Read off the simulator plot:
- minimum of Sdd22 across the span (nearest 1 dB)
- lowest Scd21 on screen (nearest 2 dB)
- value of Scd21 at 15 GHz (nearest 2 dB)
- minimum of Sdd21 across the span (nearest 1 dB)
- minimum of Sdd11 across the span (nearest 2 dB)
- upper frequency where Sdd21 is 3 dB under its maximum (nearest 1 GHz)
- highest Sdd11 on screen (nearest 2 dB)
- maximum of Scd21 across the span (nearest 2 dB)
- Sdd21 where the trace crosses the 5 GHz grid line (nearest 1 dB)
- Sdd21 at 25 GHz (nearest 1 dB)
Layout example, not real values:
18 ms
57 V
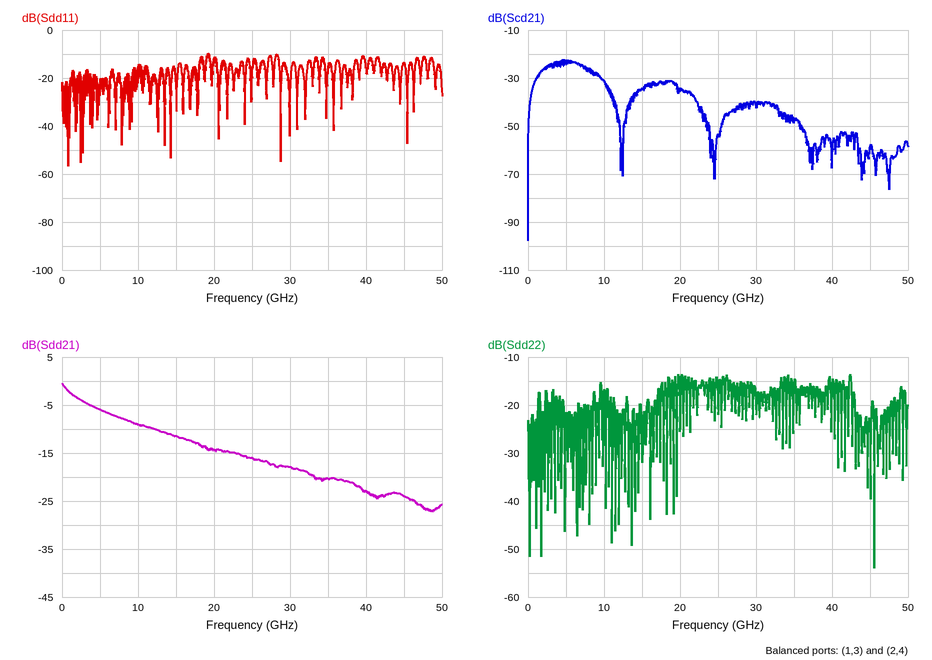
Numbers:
-54 dB
-98 dB
-34 dB
-27 dB
-56 dB
2 GHz
-10 dB
-22 dB
-6 dB
-16 dB
